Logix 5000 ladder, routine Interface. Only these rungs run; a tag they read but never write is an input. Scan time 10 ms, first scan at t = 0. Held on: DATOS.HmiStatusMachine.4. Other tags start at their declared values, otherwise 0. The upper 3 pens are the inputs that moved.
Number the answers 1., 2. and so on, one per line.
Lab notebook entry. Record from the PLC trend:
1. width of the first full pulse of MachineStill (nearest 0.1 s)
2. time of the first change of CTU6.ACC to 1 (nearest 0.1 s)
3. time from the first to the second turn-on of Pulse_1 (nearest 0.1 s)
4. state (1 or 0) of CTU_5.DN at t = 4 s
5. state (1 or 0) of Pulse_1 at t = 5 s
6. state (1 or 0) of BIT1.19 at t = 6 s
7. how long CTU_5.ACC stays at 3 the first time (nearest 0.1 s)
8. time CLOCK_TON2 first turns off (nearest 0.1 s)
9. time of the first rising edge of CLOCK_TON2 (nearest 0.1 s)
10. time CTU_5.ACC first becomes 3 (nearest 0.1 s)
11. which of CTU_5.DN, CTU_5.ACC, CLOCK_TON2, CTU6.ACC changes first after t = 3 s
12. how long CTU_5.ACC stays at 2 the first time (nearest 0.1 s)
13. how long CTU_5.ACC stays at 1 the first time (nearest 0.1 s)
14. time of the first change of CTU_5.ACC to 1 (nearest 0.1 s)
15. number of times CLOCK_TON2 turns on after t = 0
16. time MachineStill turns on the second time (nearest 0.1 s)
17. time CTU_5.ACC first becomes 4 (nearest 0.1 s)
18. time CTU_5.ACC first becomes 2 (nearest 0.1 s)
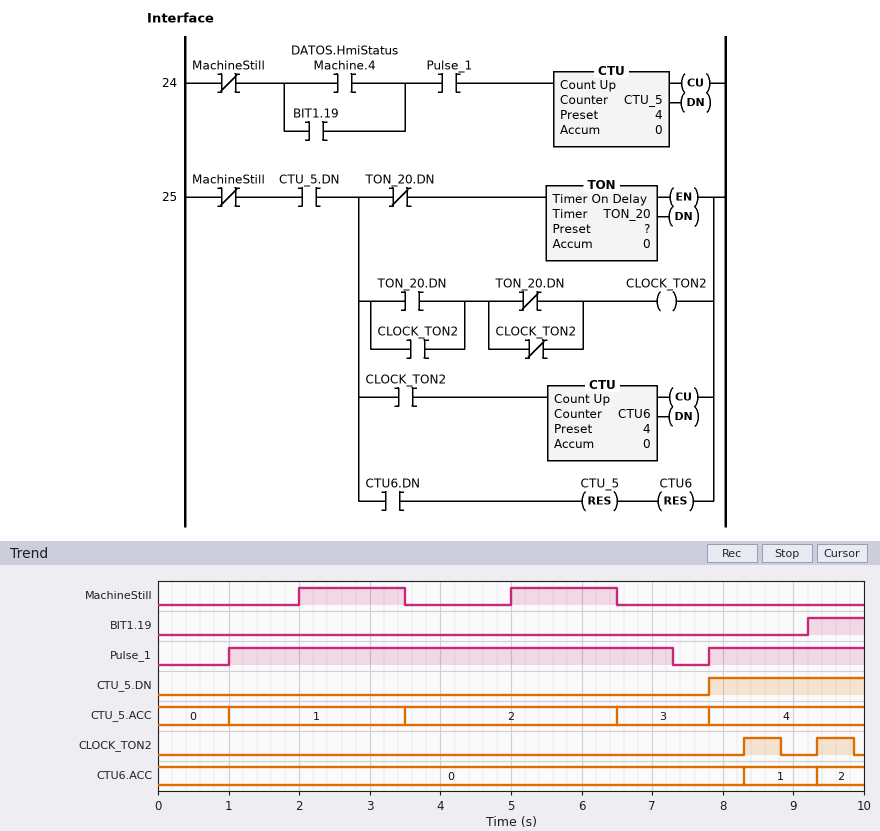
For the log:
1. 1.5 s
2. 8.3 s
3. 6.8 s
4. 0
5. 1
6. 0
7. 1.3 s
8. 8.8 s
9. 8.3 s
10. 6.5 s
11. CTU_5.ACC
12. 3.0 s
13. 2.5 s
14. 1.0 s
15. 2
16. 5.0 s
17. 7.8 s
18. 3.5 s
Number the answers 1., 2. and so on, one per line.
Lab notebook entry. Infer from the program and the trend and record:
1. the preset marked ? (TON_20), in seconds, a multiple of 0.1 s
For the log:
1. 0.5 s
